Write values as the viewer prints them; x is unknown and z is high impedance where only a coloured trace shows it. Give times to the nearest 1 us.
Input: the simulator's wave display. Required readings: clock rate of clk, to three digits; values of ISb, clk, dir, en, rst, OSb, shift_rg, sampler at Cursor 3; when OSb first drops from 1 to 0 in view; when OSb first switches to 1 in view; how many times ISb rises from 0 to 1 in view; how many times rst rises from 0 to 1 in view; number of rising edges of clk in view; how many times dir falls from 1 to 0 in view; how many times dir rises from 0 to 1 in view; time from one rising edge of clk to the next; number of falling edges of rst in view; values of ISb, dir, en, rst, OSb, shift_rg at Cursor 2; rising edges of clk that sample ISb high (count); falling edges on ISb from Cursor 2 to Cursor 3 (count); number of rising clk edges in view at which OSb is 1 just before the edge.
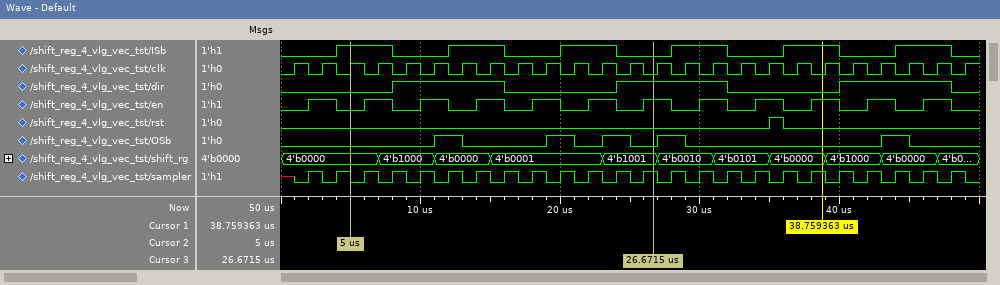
500 kHz
ISb=0, clk=0, dir=1, en=1, rst=0, OSb=0, shift_rg=4'b1001, sampler=1
13 us
11 us
6
1
25
3
3
2 us
1
ISb=1, dir=0, en=0, rst=0, OSb=0, shift_rg=4'b0000
12
3
5
